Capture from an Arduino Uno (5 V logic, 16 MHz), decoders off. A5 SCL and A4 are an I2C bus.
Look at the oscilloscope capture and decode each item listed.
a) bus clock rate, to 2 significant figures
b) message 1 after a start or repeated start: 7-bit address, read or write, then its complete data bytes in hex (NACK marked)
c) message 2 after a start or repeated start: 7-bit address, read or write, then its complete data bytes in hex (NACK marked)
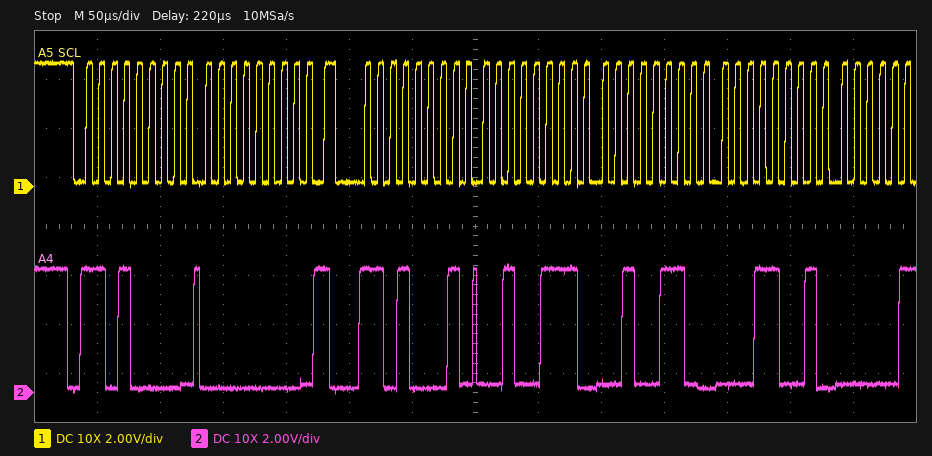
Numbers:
100 kHz
0x68 write: 00
0x68 read: 27 26 19
